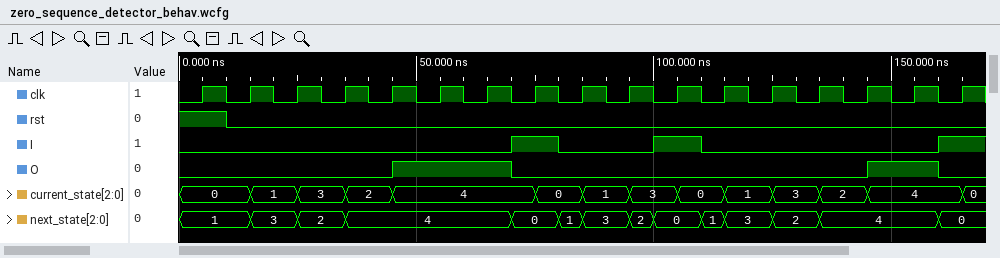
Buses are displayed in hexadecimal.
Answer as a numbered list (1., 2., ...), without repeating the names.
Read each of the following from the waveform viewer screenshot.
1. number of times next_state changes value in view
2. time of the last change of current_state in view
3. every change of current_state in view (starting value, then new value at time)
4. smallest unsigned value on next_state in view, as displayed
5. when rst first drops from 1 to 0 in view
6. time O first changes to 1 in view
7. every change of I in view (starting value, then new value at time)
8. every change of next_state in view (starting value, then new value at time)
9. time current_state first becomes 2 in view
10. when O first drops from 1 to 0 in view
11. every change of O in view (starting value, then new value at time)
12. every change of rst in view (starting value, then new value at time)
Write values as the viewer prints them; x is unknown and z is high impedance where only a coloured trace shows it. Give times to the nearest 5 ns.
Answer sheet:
1. 13
2. 165 ns
3. 0, 1 at 15 ns, 3 at 25 ns, 2 at 35 ns, 4 at 45 ns, 0 at 75 ns, 1 at 85 ns, 3 at 95 ns, 0 at 105 ns, 1 at 115 ns, 3 at 125 ns, 2 at 135 ns, 4 at 145 ns, 0 at 165 ns
4. 0
5. 10 ns
6. 45 ns
7. 0, 1 at 70 ns, 0 at 80 ns, 1 at 100 ns, 0 at 110 ns, 1 at 160 ns
8. 1, 3 at 15 ns, 2 at 25 ns, 4 at 35 ns, 0 at 70 ns, 1 at 80 ns, 3 at 85 ns, 2 at 95 ns, 0 at 100 ns, 1 at 110 ns, 3 at 115 ns, 2 at 125 ns, 4 at 135 ns, 0 at 160 ns
9. 35 ns
10. 70 ns
11. 0, 1 at 45 ns, 0 at 70 ns, 1 at 145 ns, 0 at 160 ns
12. 1, 0 at 10 ns
